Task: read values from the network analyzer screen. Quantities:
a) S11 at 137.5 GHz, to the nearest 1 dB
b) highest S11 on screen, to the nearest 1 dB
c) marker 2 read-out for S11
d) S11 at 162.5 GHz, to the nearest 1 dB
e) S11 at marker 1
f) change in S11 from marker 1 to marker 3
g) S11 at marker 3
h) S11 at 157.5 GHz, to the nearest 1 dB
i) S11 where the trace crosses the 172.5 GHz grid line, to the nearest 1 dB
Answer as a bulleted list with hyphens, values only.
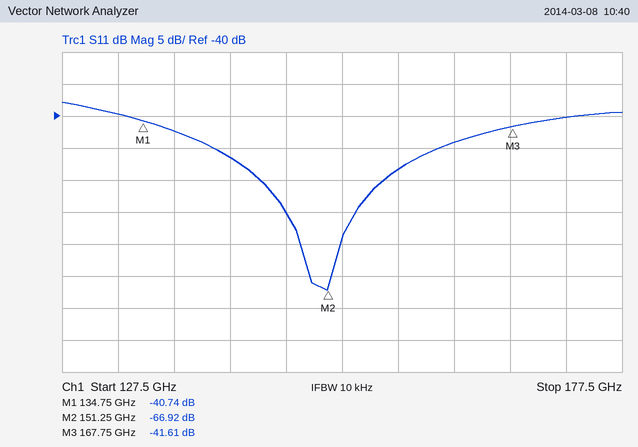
- -42 dB
- -38 dB
- -66.92 dB
- -44 dB
- -40.74 dB
- -0.87 dB
- -41.61 dB
- -48 dB
- -40 dB
